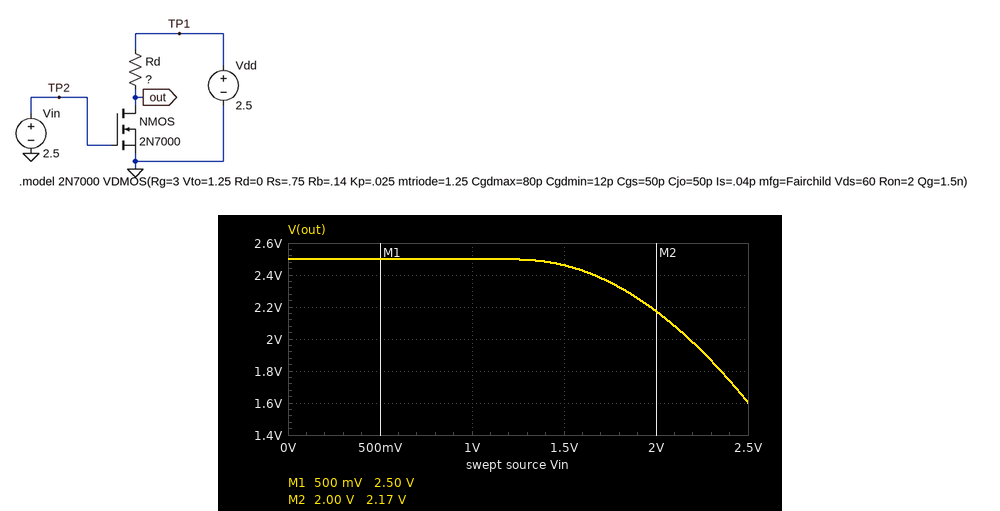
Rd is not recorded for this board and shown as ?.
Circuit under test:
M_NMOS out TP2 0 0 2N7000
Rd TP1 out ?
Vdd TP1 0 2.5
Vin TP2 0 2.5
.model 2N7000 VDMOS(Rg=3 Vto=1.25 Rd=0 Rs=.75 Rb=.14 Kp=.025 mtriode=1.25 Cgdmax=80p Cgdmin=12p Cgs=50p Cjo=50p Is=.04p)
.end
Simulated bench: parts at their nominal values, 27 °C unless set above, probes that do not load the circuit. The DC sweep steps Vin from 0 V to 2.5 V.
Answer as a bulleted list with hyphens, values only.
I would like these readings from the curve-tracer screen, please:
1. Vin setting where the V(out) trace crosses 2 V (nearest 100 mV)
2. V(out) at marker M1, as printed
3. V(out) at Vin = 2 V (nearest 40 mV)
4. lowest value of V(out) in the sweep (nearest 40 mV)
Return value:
- 2.2 V
- 2.50 V
- 2.16 V
- 1.60 V
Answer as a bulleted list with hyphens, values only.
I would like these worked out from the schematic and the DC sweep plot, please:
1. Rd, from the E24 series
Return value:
- 47 Ω
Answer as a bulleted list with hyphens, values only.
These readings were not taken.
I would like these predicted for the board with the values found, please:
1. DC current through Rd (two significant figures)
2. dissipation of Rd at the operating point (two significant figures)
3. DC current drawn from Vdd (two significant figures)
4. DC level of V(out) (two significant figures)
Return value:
- 19 mA
- 17 mW
- 19 mA
- 1.6 V
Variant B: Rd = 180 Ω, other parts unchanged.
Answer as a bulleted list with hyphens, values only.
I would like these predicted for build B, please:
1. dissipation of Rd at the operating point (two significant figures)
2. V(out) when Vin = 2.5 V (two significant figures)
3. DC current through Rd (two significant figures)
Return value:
- 25 mW
- 380 mV
- 12 mA
